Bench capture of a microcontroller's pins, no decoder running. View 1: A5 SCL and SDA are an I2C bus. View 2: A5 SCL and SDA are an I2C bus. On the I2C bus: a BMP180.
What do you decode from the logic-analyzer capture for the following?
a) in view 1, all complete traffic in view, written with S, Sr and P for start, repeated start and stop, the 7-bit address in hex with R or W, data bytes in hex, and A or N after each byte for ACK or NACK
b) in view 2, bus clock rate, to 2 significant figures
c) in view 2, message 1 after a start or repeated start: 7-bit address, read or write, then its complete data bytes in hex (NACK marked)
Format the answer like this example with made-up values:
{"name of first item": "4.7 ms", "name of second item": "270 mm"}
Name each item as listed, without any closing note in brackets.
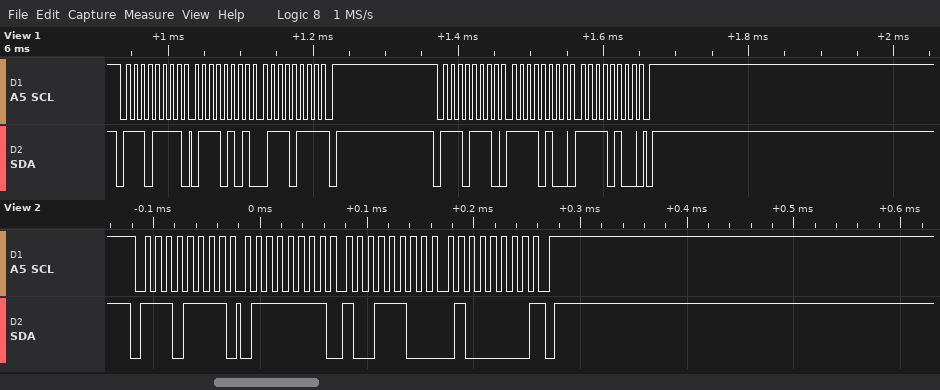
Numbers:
{"in view 1, all complete traffic in view, written with S, Sr and P for start, repeated start and stop, the 7-bit address in hex with R or W, data bytes in hex, and A or N after each byte for ACK or NACK": "S 77R A 75 A 77 N P S 77W A F4 A F4 A P", "in view 2, bus clock rate, to 2 significant figures": "100 kHz", "in view 2, message 1 after a start or repeated start: 7-bit address, read or write, then its complete data bytes in hex": "0x77 read: 7F 9C 40 NACK"}
